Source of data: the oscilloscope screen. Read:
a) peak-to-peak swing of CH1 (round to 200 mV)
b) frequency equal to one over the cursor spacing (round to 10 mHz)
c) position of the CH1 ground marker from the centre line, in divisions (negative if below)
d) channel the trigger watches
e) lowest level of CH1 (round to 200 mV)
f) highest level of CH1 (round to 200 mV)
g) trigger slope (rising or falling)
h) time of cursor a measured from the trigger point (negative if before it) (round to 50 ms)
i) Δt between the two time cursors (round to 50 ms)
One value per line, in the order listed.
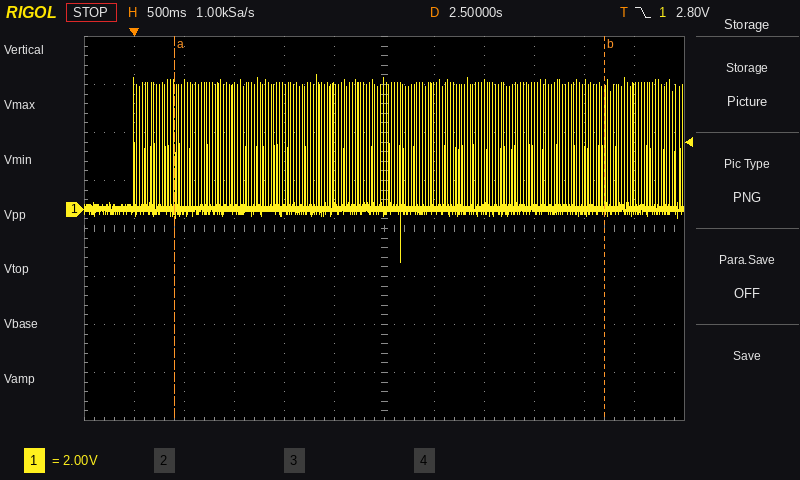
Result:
7.8 V
230 mHz
+0.4 div
CH1
-2.2 V
5.6 V
falling
+400 ms
4.30 s
